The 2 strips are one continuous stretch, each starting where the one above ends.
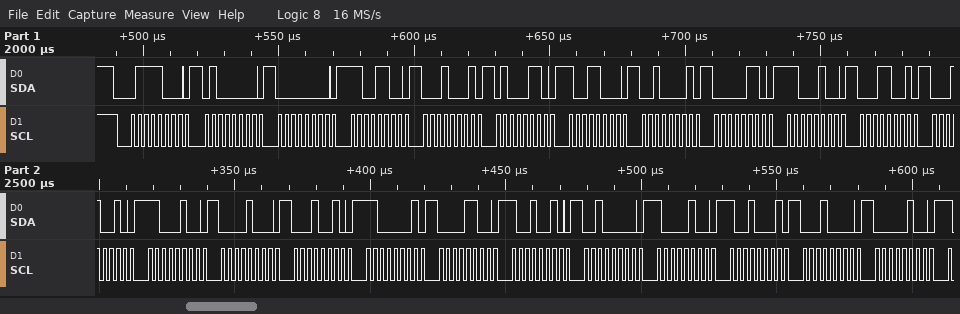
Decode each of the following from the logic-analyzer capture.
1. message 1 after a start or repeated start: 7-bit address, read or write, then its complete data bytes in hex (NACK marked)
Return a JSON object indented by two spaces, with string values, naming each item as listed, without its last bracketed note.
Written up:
{
  "message 1 after a start or repeated start: 7-bit address, read or write, then its complete data bytes in hex": "0x3C write: 40 00 CC 11 46 98 21 06 C4 19 12 C4 08 12 C1 0C 92 20 84 91 10 04"
}
